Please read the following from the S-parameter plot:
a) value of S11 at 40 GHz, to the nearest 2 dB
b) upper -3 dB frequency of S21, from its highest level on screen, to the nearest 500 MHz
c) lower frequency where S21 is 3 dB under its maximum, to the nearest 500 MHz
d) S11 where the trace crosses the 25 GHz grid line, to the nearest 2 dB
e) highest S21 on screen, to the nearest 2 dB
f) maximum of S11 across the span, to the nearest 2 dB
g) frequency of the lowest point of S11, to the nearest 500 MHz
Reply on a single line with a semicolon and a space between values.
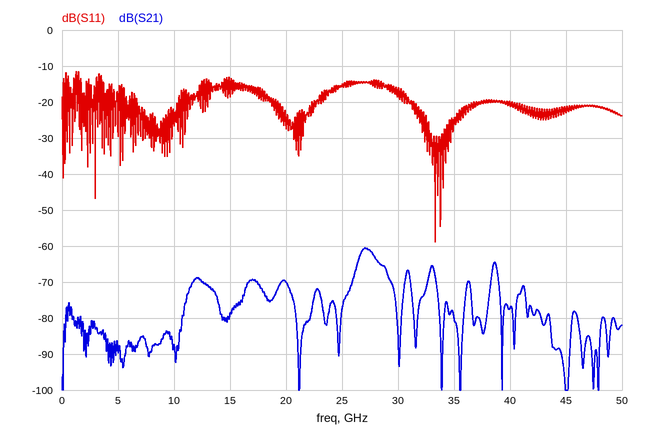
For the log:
-20 dB; 28.0 GHz; 26.5 GHz; -16 dB; -60 dB; -12 dB; 33.5 GHz
